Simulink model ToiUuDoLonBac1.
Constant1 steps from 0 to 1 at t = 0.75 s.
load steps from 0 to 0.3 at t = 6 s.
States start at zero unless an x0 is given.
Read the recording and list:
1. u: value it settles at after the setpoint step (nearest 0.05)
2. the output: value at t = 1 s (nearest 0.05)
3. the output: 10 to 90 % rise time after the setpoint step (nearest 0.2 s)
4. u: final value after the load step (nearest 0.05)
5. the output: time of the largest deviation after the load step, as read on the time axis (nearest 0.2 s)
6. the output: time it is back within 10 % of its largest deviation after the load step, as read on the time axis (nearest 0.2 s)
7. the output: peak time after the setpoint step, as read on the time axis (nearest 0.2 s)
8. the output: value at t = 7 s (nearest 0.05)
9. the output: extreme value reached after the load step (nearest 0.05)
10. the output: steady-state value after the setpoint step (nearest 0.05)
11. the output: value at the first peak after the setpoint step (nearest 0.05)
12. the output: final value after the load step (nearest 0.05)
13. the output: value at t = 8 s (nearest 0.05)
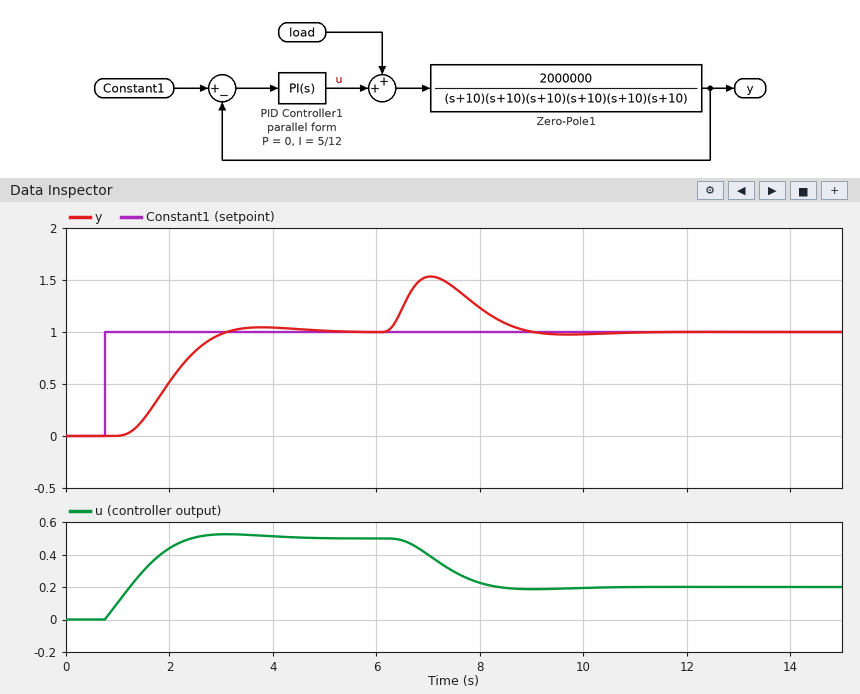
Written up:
0.50
0.00
1.4 s
0.20
7.0 s
8.6 s
3.8 s
1.55
1.55
1.00
1.05
1.00
1.25
